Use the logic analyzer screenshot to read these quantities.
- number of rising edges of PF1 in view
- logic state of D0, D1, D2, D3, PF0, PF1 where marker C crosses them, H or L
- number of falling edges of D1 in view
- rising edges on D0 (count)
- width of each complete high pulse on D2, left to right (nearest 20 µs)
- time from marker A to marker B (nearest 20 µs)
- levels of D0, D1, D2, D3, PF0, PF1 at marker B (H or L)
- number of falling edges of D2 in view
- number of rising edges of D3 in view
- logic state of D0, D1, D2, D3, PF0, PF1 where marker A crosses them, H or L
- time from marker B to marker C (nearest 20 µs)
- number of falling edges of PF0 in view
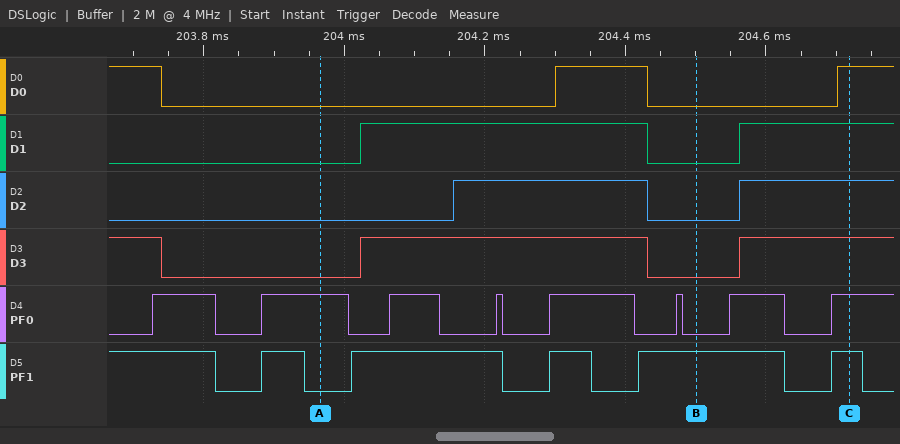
5
D0=H, D1=H, D2=H, D3=H, PF0=H, PF1=H
1
2
280 µs
540 µs
D0=L, D1=L, D2=L, D3=L, PF0=L, PF1=H
1
2
D0=L, D1=L, D2=L, D3=L, PF0=H, PF1=L
220 µs
7
